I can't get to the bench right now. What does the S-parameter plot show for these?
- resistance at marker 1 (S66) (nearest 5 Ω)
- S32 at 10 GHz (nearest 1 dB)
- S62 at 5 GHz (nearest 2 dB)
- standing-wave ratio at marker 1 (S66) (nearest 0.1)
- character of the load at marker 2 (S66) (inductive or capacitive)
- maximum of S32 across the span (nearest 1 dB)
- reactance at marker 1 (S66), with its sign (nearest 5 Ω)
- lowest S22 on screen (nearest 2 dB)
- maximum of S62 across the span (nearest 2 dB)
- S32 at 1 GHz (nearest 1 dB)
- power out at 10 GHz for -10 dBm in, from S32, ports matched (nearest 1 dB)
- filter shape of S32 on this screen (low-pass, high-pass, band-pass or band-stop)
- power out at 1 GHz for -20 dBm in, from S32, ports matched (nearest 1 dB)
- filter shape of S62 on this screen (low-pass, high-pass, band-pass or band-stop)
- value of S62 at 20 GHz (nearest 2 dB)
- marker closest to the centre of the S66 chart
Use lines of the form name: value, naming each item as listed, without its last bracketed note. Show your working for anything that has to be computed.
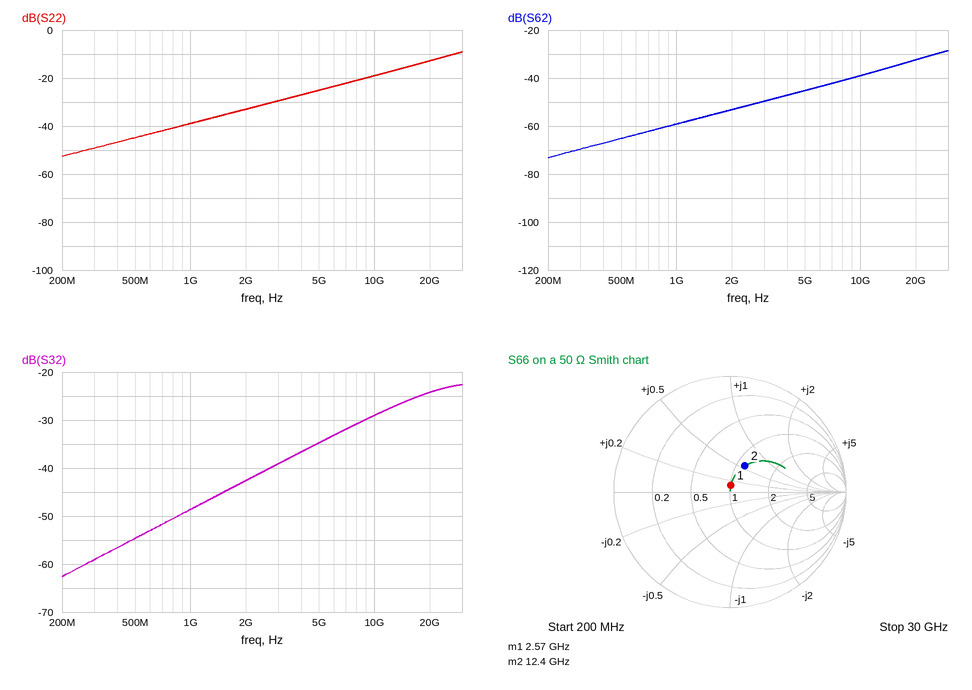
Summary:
resistance at marker 1 (S66): 50 Ω
S32 at 10 GHz: -29 dB
S62 at 5 GHz: -46 dB
standing-wave ratio at marker 1 (S66): 1.1
character of the load at marker 2 (S66): inductive
maximum of S32 across the span: -23 dB
reactance at marker 1 (S66), with its sign: +5 Ω
lowest S22 on screen: -52 dB
maximum of S62 across the span: -28 dB
S32 at 1 GHz: -49 dB
power out at 10 GHz for -10 dBm in, from S32, ports matched: -10 dBm + (-29 dB) = -39 dBm
filter shape of S32 on this screen: high-pass
power out at 1 GHz for -20 dBm in, from S32, ports matched: -20 dBm + (-49 dB) = -69 dBm
filter shape of S62 on this screen: high-pass
value of S62 at 20 GHz: -32 dB
marker closest to the centre of the S66 chart: marker 1
